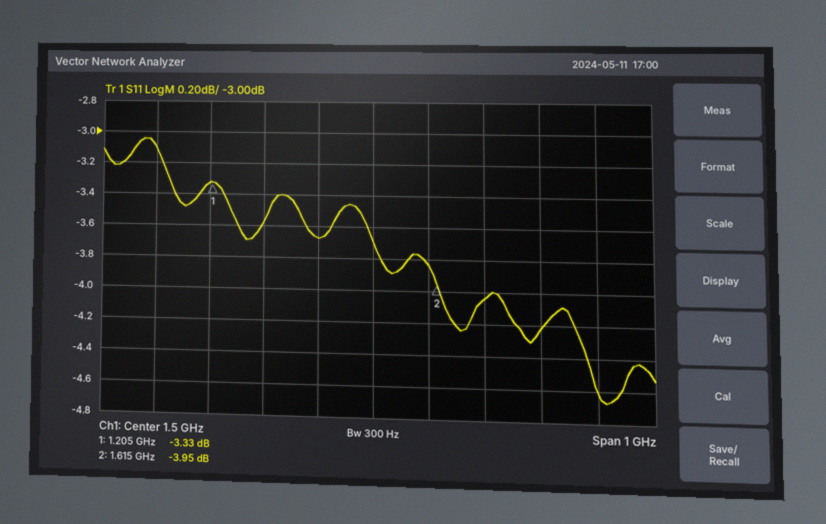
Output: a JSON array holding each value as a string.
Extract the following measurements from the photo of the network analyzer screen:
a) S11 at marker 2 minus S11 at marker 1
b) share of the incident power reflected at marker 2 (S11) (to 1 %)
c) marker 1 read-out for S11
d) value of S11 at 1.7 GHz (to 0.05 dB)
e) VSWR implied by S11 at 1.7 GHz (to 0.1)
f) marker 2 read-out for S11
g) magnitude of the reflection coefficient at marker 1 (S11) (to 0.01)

["-0.62 dB", "40 %", "-3.33 dB", "-4.05 dB", "4.4", "-3.95 dB", "0.68"]
